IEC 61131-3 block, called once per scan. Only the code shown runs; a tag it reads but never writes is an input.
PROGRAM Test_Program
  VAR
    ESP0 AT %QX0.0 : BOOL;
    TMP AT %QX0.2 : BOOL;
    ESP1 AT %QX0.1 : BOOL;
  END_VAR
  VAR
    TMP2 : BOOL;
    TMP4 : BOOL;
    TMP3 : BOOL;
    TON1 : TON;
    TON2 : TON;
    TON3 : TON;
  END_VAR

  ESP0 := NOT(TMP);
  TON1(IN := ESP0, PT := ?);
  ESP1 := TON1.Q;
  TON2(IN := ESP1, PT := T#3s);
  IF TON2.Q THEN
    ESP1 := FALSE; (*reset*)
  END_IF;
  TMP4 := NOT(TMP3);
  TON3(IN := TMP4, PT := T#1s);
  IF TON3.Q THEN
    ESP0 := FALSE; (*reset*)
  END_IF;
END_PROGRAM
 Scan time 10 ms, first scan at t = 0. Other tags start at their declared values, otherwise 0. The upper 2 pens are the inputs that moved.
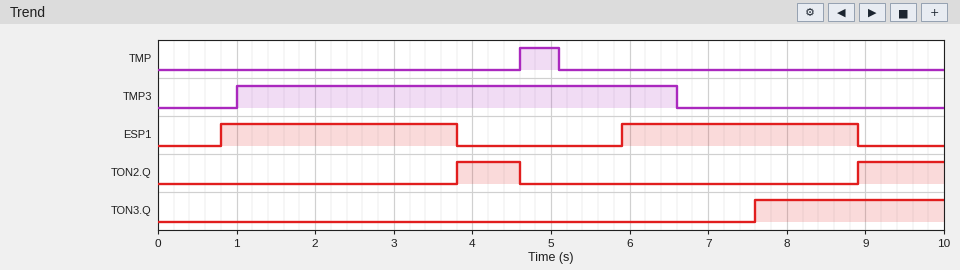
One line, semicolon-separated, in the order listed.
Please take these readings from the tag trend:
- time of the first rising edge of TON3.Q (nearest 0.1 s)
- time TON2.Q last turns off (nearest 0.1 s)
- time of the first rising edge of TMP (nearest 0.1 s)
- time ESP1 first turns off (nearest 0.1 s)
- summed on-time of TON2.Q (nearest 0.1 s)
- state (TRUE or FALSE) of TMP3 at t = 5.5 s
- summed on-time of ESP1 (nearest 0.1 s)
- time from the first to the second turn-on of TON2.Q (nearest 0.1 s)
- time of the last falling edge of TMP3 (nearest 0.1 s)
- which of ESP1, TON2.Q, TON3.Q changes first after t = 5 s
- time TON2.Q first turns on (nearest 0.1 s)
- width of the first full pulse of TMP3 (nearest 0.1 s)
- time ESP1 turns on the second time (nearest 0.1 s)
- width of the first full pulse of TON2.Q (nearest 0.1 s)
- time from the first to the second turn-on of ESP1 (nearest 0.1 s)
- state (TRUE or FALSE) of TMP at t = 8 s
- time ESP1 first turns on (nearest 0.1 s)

7.6 s; 4.6 s; 4.6 s; 3.8 s; 1.9 s; TRUE; 6.0 s; 5.1 s; 6.6 s; ESP1; 3.8 s; 5.6 s; 5.9 s; 0.8 s; 5.1 s; FALSE; 0.8 s
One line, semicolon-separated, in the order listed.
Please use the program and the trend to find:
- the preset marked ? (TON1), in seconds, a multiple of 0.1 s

0.8 s
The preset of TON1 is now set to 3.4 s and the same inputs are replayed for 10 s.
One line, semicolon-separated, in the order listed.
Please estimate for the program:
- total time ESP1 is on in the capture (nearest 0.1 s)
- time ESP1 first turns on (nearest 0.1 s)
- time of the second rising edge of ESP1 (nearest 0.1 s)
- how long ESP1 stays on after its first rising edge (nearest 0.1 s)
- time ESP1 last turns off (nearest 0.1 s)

2.7 s; 3.4 s; 8.5 s; 1.2 s; 4.6 s
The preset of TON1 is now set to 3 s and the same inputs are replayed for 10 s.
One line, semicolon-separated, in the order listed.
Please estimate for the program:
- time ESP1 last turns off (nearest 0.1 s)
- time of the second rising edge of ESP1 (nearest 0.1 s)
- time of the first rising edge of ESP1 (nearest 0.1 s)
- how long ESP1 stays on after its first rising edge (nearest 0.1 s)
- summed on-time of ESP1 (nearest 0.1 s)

4.6 s; 8.1 s; 3.0 s; 1.6 s; 3.5 s
